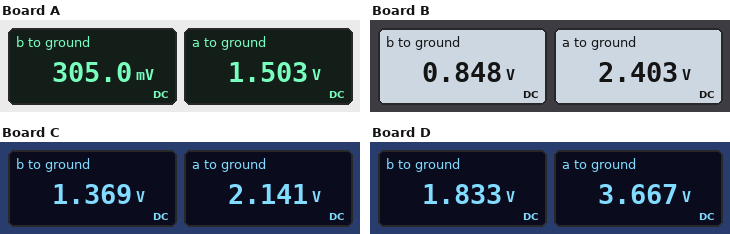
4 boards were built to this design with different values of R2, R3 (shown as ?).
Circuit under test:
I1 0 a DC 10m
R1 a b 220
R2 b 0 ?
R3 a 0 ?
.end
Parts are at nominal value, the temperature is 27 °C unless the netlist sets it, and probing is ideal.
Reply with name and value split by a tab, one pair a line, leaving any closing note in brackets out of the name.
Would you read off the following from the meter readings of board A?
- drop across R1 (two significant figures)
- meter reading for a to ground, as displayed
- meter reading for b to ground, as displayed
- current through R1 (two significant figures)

drop across R1	1.2 V
meter reading for a to ground, as displayed	1.503 V
meter reading for b to ground, as displayed	305.0 mV
current through R1	5.4 mA
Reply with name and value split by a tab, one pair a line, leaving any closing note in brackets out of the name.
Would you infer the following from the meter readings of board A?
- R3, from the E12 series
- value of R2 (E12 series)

R3, from the E12 series	330 Ω
value of R2	56 Ω
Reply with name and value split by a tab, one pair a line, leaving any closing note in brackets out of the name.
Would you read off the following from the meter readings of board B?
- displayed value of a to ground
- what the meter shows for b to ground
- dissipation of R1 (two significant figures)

displayed value of a to ground	2.403 V
what the meter shows for b to ground	0.848 V
dissipation of R1	11 mW
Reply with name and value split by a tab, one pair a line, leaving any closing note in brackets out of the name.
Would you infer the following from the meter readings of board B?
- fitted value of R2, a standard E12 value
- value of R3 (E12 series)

fitted value of R2, a standard E12 value	120 Ω
value of R3	820 Ω
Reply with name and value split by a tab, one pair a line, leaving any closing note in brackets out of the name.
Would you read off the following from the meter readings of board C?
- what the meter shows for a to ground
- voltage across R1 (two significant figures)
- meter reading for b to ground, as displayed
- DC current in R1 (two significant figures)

what the meter shows for a to ground	2.141 V
voltage across R1	770 mV
meter reading for b to ground, as displayed	1.369 V
DC current in R1	3.5 mA
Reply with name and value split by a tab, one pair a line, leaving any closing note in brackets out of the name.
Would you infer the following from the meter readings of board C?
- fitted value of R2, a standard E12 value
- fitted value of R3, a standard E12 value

fitted value of R2, a standard E12 value	390 Ω
fitted value of R3, a standard E12 value	330 Ω
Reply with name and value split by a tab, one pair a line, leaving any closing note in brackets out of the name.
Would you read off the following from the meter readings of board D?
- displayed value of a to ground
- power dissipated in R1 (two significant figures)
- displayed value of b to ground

displayed value of a to ground	3.667 V
power dissipated in R1	15 mW
displayed value of b to ground	1.833 V
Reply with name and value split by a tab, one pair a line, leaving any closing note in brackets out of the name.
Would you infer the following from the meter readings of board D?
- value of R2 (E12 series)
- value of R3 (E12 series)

value of R2	220 Ω
value of R3	2.2 kΩ
